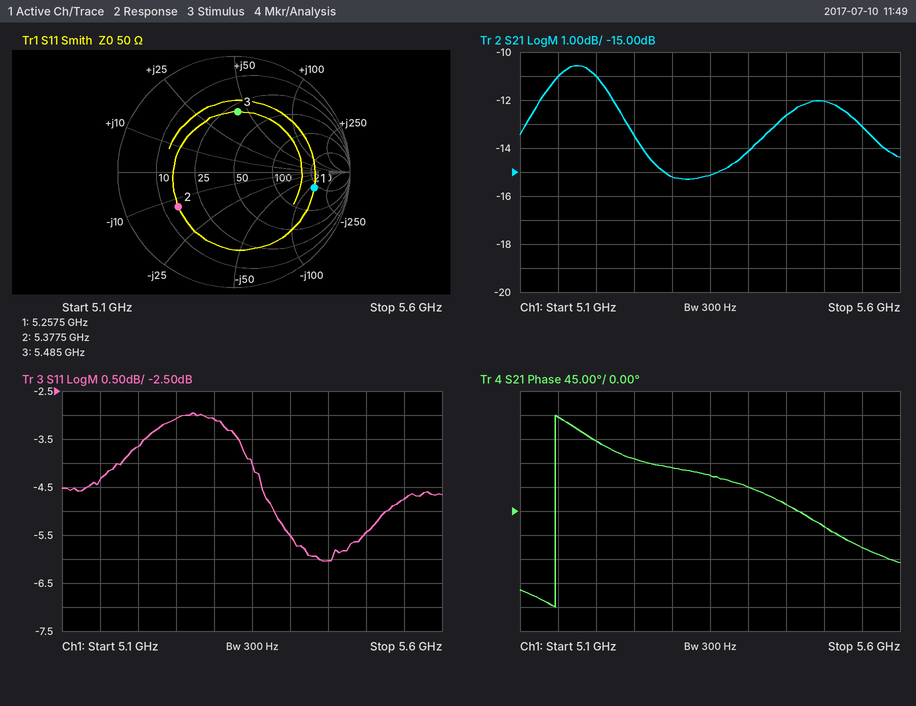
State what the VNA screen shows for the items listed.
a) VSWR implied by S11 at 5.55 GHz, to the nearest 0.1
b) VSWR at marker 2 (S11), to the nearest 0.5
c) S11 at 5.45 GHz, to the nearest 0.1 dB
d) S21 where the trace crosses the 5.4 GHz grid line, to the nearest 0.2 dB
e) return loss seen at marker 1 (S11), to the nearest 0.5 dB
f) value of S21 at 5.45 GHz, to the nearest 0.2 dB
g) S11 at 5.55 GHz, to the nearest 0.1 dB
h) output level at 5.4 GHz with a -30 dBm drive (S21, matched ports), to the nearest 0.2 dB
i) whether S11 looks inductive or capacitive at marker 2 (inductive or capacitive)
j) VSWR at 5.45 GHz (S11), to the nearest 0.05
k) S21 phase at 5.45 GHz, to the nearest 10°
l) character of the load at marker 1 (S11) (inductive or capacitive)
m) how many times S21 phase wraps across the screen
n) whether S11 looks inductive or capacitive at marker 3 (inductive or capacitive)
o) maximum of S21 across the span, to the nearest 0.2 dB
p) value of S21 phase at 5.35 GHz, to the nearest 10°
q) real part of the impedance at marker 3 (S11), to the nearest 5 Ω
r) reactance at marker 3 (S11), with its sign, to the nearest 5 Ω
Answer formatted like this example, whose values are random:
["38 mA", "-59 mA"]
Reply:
["3.7", "3.5", "-6.0 dB", "-14.2 dB", "3.0 dB", "-12.6 dB", "-4.8 dB", "-44.2 dBm", "capacitive", "3.00", "10°", "capacitive", "1", "inductive", "-10.6 dB", "70°", "30 Ω", "+45 Ω"]
